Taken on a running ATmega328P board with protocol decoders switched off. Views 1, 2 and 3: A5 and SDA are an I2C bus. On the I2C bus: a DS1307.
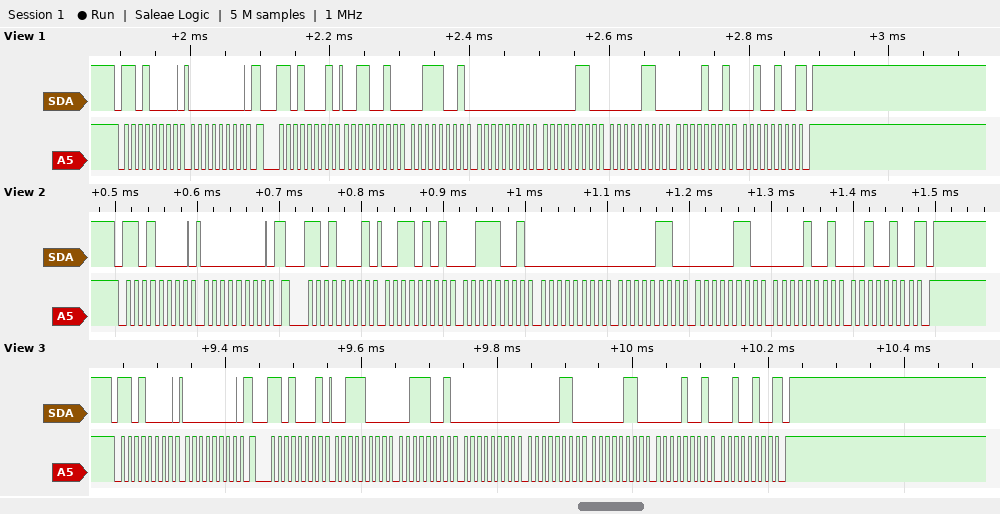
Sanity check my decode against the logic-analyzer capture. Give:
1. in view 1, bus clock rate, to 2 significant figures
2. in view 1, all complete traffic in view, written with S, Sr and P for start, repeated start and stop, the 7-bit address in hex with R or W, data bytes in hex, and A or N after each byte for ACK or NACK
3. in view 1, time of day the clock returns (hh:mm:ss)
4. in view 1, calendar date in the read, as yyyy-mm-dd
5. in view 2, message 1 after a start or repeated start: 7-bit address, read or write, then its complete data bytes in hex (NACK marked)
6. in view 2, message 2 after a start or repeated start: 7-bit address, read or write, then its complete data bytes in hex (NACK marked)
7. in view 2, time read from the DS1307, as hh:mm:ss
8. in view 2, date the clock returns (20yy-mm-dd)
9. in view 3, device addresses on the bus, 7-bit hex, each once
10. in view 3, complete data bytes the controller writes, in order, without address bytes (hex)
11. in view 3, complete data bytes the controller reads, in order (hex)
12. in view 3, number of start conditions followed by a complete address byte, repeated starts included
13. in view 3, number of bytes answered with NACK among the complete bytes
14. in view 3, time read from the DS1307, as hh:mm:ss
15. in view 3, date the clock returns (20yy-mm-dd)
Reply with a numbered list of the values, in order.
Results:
1. 100 kHz
2. S 68W A 00 A Sr 68R A 32 A 39 A 00 A 06 A 06 A 09 A 24 N P
3. 00:39:32
4. 2024-09-06
5. 0x68 write: 00
6. 0x68 read: 35 39 00 06 06 09 24 NACK
7. 00:39:35
8. 2024-09-06
9. 0x68
10. 00
11. 38 39 00 06 06 09 24
12. 2
13. 1
14. 00:39:38
15. 2024-09-06
